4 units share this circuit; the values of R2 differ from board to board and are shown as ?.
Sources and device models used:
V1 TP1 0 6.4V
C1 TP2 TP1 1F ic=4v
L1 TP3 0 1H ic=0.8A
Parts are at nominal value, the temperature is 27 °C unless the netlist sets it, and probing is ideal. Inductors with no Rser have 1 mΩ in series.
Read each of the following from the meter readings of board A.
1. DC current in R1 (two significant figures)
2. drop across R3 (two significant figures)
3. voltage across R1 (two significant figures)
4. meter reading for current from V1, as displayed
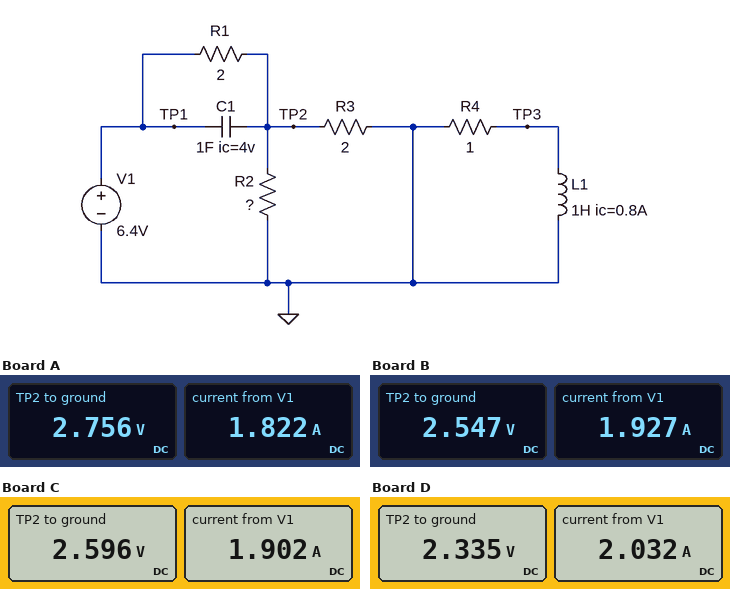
1.8 A
2.8 V
3.6 V
1.822 A
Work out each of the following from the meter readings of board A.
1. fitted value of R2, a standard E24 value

6.2 Ω
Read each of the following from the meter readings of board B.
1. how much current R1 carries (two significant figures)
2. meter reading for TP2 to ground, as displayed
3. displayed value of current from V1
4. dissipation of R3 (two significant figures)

1.9 A
2.547 V
1.927 A
3.2 W
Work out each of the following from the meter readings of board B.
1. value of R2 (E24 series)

3.9 Ω
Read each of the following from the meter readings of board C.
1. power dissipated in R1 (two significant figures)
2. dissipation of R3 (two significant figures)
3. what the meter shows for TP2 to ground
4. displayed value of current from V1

7.2 W
3.4 W
2.596 V
1.902 A
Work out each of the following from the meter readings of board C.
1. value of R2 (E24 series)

4.3 Ω
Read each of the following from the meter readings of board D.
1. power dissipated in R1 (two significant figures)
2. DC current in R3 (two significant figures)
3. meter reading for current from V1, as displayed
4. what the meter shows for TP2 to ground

8.3 W
1.2 A
2.032 A
2.335 V
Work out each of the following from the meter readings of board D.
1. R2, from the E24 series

2.7 Ω
